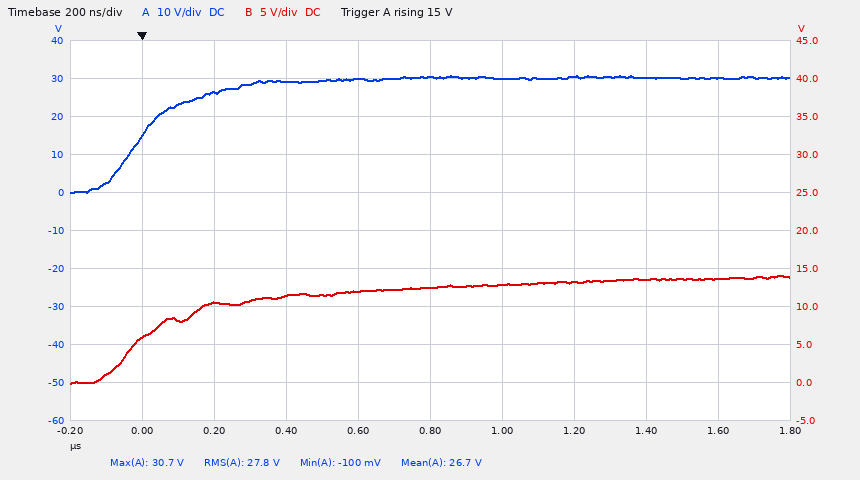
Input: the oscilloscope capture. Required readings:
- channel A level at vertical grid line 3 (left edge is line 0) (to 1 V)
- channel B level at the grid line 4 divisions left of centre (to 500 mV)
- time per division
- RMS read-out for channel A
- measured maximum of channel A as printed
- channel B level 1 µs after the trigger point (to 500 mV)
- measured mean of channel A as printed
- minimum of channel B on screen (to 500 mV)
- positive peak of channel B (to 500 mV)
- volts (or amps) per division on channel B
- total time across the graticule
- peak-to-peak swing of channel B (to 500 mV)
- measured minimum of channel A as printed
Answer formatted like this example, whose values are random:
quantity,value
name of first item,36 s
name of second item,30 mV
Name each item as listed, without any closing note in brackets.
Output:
quantity,value
channel A level at vertical grid line 3 (left edge is line 0),29 V
channel B level at the grid line 4 divisions left of centre,6.0 V
time per division,200 ns
RMS read-out for channel A,27.8 V
measured maximum of channel A as printed,30.7 V
channel B level 1 µs after the trigger point,13.0 V
measured mean of channel A as printed,26.7 V
minimum of channel B on screen,0.0 V
positive peak of channel B,14.0 V
volts (or amps) per division on channel B,5 V
total time across the graticule,2 µs
peak-to-peak swing of channel B,14.0 V
measured minimum of channel A as printed,-100 mV
